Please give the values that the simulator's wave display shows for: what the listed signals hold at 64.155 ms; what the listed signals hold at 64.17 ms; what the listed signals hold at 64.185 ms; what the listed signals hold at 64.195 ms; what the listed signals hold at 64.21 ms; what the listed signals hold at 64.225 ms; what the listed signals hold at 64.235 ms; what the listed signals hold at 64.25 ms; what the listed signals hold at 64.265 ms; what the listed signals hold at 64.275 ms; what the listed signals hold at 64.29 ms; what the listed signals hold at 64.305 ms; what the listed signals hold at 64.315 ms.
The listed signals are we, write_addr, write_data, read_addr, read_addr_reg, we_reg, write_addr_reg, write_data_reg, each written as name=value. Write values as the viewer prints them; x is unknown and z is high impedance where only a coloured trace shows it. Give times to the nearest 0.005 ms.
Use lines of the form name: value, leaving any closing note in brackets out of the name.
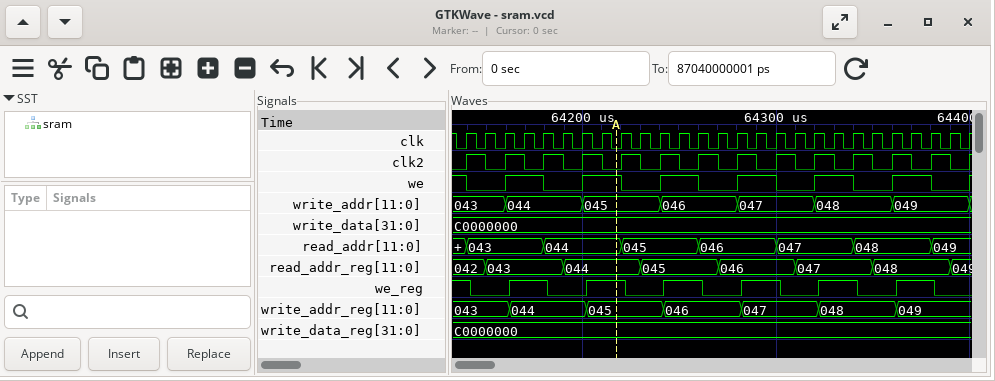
what the listed signals hold at 64.155 ms: we=0, write_addr=043, write_data=C0000000, read_addr=043, read_addr_reg=043, we_reg=0, write_addr_reg=043, write_data_reg=C0000000
what the listed signals hold at 64.17 ms: we=1, write_addr=044, write_data=C0000000, read_addr=043, read_addr_reg=043, we_reg=1, write_addr_reg=044, write_data_reg=C0000000
what the listed signals hold at 64.185 ms: we=0, write_addr=044, write_data=C0000000, read_addr=044, read_addr_reg=043, we_reg=0, write_addr_reg=044, write_data_reg=C0000000
what the listed signals hold at 64.195 ms: we=0, write_addr=044, write_data=C0000000, read_addr=044, read_addr_reg=044, we_reg=0, write_addr_reg=044, write_data_reg=C0000000
what the listed signals hold at 64.21 ms: we=1, write_addr=045, write_data=C0000000, read_addr=044, read_addr_reg=044, we_reg=1, write_addr_reg=045, write_data_reg=C0000000
what the listed signals hold at 64.225 ms: we=0, write_addr=045, write_data=C0000000, read_addr=045, read_addr_reg=044, we_reg=0, write_addr_reg=045, write_data_reg=C0000000
what the listed signals hold at 64.235 ms: we=0, write_addr=045, write_data=C0000000, read_addr=045, read_addr_reg=045, we_reg=0, write_addr_reg=045, write_data_reg=C0000000
what the listed signals hold at 64.25 ms: we=1, write_addr=046, write_data=C0000000, read_addr=045, read_addr_reg=045, we_reg=1, write_addr_reg=046, write_data_reg=C0000000
what the listed signals hold at 64.265 ms: we=0, write_addr=046, write_data=C0000000, read_addr=046, read_addr_reg=045, we_reg=0, write_addr_reg=046, write_data_reg=C0000000
what the listed signals hold at 64.275 ms: we=0, write_addr=046, write_data=C0000000, read_addr=046, read_addr_reg=046, we_reg=0, write_addr_reg=046, write_data_reg=C0000000
what the listed signals hold at 64.29 ms: we=1, write_addr=047, write_data=C0000000, read_addr=046, read_addr_reg=046, we_reg=1, write_addr_reg=047, write_data_reg=C0000000
what the listed signals hold at 64.305 ms: we=0, write_addr=047, write_data=C0000000, read_addr=047, read_addr_reg=046, we_reg=0, write_addr_reg=047, write_data_reg=C0000000
what the listed signals hold at 64.315 ms: we=0, write_addr=047, write_data=C0000000, read_addr=047, read_addr_reg=047, we_reg=0, write_addr_reg=047, write_data_reg=C0000000
